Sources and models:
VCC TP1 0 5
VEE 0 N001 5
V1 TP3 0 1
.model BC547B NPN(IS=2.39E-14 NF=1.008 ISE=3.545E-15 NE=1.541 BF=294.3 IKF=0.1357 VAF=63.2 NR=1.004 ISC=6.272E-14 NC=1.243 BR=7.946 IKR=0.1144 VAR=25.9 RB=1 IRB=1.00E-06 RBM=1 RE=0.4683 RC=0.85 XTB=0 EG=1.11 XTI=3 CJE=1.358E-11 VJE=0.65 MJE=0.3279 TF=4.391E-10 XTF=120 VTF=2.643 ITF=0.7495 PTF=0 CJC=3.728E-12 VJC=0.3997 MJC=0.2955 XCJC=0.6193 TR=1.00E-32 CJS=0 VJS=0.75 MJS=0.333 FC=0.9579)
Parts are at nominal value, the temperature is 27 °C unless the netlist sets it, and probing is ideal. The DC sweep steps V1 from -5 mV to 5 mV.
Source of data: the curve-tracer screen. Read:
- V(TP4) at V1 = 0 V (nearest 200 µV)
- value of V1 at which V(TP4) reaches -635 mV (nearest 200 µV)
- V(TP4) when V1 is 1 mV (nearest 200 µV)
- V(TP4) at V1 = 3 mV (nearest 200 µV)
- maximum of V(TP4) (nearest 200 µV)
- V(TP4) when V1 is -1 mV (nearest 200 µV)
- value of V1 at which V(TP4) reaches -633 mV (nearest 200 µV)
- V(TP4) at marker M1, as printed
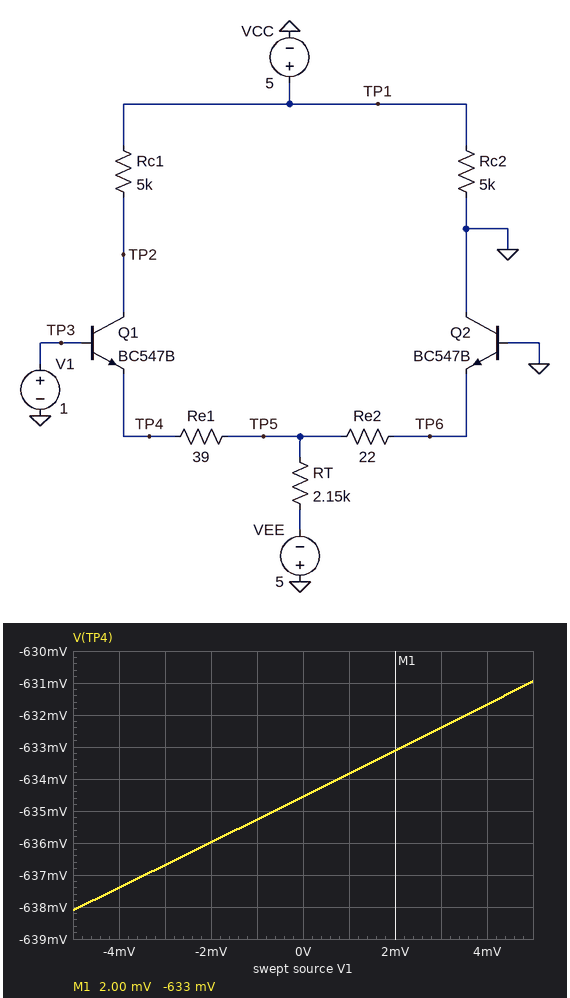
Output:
-634.6 mV
-600 µV
-633.8 mV
-632.4 mV
-631.0 mV
-635.2 mV
2.2 mV
-633 mV
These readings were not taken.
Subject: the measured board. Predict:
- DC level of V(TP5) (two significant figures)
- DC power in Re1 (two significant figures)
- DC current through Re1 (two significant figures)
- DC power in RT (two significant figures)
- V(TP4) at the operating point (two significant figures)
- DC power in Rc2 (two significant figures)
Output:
200 mV
230 µW
2.4 mA
13 mW
290 mV
5.0 mW
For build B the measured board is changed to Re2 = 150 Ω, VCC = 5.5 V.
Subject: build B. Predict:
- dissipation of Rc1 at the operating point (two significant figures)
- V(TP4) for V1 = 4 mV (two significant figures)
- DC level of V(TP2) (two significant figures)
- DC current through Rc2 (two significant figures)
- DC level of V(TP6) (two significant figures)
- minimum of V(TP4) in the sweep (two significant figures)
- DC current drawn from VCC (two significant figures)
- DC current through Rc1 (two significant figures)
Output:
5.4 mW
-660 mV
310 mV
1.1 mA
200 mV
-670 mV
2.1 mA
1.0 mA
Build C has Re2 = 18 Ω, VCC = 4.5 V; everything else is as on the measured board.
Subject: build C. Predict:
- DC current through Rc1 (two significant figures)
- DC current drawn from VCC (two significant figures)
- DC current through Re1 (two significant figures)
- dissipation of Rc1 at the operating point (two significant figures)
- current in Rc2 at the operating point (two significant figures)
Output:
840 µA
1.7 mA
2.4 mA
3.5 mW
900 µA
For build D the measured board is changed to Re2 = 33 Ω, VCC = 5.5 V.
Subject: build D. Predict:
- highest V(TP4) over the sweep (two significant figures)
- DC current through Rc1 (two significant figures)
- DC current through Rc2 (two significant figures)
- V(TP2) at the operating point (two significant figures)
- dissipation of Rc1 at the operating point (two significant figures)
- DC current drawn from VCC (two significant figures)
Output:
-630 mV
1.0 mA
1.1 mA
310 mV
5.4 mW
2.1 mA
